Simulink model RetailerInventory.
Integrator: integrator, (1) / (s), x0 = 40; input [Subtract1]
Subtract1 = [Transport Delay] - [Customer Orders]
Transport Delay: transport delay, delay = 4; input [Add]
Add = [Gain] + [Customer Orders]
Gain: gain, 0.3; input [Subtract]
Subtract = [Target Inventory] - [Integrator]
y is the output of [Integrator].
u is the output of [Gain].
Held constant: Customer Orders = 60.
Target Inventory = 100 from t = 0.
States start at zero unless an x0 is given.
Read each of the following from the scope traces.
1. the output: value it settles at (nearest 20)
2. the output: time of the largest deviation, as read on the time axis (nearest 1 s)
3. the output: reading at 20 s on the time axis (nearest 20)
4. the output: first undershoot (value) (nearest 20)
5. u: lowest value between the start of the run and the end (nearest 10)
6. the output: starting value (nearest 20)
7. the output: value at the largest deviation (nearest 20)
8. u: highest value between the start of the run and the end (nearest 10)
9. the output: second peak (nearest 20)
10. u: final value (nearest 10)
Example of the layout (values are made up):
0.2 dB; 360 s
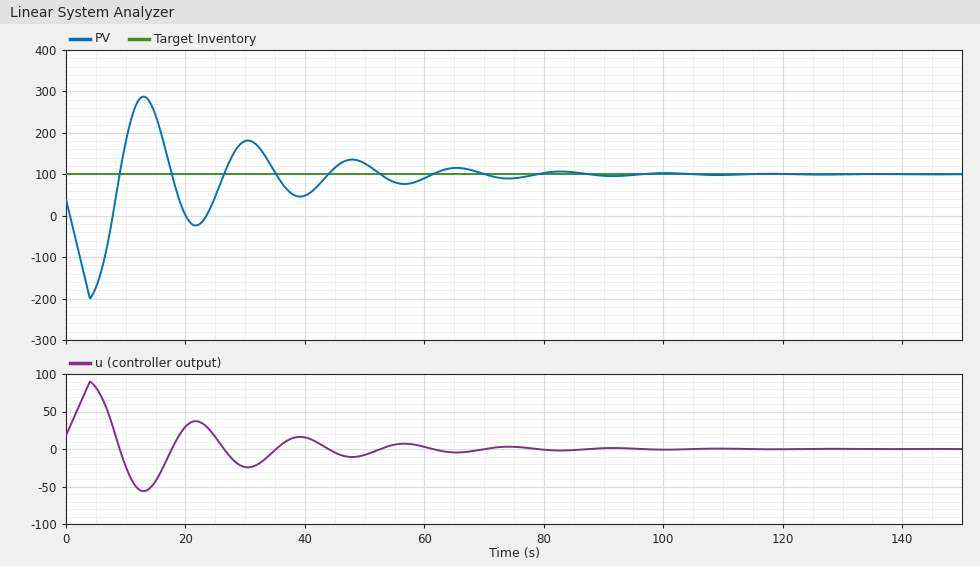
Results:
100; 13 s; 0; -20; -60; 40; 280; 90; 180; 0
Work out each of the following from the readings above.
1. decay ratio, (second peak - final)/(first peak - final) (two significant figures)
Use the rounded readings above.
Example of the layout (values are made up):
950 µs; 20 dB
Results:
0.44
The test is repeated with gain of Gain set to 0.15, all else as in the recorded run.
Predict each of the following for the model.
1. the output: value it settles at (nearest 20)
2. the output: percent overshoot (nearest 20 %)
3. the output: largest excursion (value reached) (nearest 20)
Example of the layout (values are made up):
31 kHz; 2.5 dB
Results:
100; 60 %; 140
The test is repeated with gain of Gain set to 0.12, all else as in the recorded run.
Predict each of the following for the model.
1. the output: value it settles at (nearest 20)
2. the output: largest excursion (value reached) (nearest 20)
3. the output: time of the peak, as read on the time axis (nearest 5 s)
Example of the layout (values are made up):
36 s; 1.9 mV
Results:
100; 100; 20 s
